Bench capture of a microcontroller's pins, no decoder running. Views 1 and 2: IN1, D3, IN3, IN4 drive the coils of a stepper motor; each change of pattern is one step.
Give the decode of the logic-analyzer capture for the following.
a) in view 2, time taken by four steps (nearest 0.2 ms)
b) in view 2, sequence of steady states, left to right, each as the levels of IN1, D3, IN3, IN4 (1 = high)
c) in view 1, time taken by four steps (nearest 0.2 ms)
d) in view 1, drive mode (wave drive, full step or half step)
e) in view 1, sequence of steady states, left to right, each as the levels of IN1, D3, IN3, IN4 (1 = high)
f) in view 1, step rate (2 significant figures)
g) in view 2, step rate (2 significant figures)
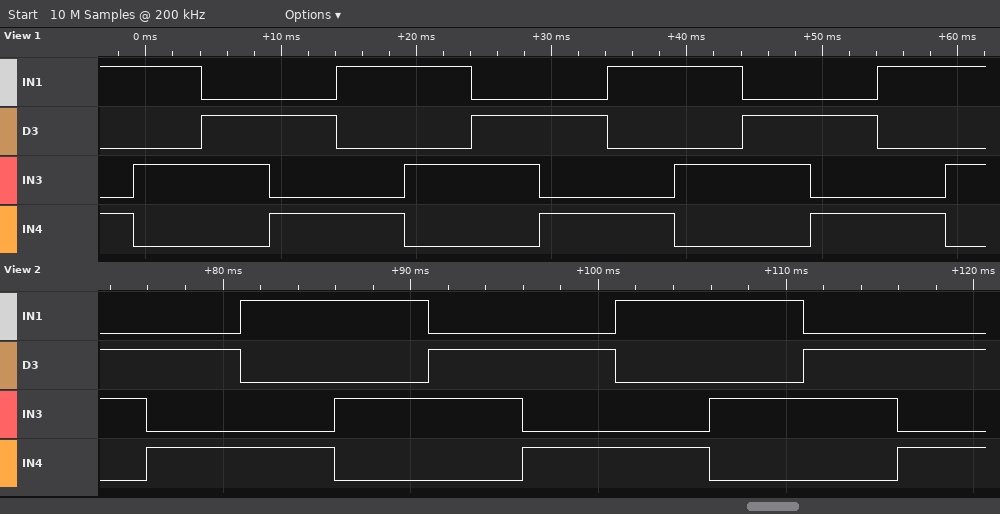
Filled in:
20.0 ms
0110 0101 1001 1010 0110 0101 1001 1010 0110 0101
20.0 ms
full step
1001 1010 0110 0101 1001 1010 0110 0101 1001 1010 0110 0101 1001 1010
200 steps/s
200 steps/s
